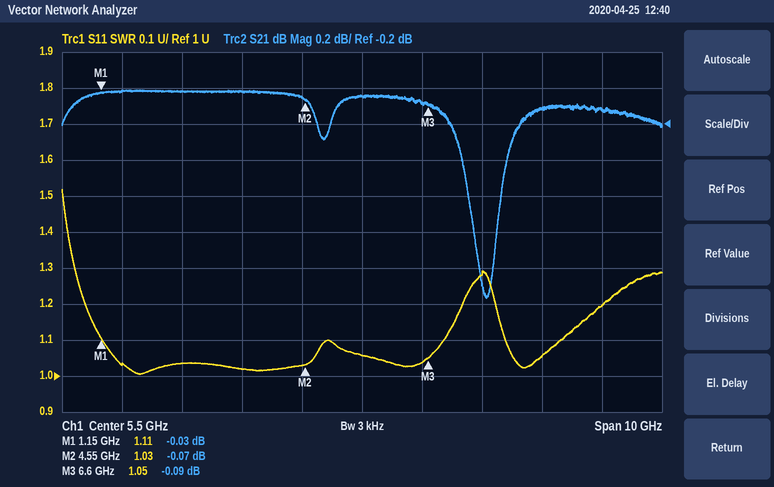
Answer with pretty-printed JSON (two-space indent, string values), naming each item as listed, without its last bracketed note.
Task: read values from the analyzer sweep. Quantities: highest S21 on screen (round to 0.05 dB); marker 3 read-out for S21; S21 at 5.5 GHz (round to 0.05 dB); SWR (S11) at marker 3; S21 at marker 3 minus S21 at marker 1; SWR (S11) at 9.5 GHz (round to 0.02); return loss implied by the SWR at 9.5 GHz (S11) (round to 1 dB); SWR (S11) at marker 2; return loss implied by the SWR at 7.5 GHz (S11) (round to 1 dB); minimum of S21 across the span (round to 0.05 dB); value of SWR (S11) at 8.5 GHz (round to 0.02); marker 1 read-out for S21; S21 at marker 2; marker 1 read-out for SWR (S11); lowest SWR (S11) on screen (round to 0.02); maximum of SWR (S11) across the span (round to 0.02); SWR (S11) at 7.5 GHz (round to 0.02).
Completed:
{
  "highest S21 on screen": "0.00 dB",
  "marker 3 read-out for S21": "-0.09 dB",
  "S21 at 5.5 GHz": "-0.05 dB",
  "SWR (S11) at marker 3": "1.05",
  "S21 at marker 3 minus S21 at marker 1": "-0.06 dB",
  "SWR (S11) at 9.5 GHz": "1.20",
  "return loss implied by the SWR at 9.5 GHz (S11)": "21 dB",
  "SWR (S11) at marker 2": "1.03",
  "return loss implied by the SWR at 7.5 GHz (S11)": "18 dB",
  "minimum of S21 across the span": "-1.15 dB",
  "value of SWR (S11) at 8.5 GHz": "1.06",
  "marker 1 read-out for S21": "-0.03 dB",
  "S21 at marker 2": "-0.07 dB",
  "marker 1 read-out for SWR": "1.11",
  "lowest SWR (S11) on screen": "1.00",
  "maximum of SWR (S11) across the span": "1.52",
  "SWR (S11) at 7.5 GHz": "1.28"
}
